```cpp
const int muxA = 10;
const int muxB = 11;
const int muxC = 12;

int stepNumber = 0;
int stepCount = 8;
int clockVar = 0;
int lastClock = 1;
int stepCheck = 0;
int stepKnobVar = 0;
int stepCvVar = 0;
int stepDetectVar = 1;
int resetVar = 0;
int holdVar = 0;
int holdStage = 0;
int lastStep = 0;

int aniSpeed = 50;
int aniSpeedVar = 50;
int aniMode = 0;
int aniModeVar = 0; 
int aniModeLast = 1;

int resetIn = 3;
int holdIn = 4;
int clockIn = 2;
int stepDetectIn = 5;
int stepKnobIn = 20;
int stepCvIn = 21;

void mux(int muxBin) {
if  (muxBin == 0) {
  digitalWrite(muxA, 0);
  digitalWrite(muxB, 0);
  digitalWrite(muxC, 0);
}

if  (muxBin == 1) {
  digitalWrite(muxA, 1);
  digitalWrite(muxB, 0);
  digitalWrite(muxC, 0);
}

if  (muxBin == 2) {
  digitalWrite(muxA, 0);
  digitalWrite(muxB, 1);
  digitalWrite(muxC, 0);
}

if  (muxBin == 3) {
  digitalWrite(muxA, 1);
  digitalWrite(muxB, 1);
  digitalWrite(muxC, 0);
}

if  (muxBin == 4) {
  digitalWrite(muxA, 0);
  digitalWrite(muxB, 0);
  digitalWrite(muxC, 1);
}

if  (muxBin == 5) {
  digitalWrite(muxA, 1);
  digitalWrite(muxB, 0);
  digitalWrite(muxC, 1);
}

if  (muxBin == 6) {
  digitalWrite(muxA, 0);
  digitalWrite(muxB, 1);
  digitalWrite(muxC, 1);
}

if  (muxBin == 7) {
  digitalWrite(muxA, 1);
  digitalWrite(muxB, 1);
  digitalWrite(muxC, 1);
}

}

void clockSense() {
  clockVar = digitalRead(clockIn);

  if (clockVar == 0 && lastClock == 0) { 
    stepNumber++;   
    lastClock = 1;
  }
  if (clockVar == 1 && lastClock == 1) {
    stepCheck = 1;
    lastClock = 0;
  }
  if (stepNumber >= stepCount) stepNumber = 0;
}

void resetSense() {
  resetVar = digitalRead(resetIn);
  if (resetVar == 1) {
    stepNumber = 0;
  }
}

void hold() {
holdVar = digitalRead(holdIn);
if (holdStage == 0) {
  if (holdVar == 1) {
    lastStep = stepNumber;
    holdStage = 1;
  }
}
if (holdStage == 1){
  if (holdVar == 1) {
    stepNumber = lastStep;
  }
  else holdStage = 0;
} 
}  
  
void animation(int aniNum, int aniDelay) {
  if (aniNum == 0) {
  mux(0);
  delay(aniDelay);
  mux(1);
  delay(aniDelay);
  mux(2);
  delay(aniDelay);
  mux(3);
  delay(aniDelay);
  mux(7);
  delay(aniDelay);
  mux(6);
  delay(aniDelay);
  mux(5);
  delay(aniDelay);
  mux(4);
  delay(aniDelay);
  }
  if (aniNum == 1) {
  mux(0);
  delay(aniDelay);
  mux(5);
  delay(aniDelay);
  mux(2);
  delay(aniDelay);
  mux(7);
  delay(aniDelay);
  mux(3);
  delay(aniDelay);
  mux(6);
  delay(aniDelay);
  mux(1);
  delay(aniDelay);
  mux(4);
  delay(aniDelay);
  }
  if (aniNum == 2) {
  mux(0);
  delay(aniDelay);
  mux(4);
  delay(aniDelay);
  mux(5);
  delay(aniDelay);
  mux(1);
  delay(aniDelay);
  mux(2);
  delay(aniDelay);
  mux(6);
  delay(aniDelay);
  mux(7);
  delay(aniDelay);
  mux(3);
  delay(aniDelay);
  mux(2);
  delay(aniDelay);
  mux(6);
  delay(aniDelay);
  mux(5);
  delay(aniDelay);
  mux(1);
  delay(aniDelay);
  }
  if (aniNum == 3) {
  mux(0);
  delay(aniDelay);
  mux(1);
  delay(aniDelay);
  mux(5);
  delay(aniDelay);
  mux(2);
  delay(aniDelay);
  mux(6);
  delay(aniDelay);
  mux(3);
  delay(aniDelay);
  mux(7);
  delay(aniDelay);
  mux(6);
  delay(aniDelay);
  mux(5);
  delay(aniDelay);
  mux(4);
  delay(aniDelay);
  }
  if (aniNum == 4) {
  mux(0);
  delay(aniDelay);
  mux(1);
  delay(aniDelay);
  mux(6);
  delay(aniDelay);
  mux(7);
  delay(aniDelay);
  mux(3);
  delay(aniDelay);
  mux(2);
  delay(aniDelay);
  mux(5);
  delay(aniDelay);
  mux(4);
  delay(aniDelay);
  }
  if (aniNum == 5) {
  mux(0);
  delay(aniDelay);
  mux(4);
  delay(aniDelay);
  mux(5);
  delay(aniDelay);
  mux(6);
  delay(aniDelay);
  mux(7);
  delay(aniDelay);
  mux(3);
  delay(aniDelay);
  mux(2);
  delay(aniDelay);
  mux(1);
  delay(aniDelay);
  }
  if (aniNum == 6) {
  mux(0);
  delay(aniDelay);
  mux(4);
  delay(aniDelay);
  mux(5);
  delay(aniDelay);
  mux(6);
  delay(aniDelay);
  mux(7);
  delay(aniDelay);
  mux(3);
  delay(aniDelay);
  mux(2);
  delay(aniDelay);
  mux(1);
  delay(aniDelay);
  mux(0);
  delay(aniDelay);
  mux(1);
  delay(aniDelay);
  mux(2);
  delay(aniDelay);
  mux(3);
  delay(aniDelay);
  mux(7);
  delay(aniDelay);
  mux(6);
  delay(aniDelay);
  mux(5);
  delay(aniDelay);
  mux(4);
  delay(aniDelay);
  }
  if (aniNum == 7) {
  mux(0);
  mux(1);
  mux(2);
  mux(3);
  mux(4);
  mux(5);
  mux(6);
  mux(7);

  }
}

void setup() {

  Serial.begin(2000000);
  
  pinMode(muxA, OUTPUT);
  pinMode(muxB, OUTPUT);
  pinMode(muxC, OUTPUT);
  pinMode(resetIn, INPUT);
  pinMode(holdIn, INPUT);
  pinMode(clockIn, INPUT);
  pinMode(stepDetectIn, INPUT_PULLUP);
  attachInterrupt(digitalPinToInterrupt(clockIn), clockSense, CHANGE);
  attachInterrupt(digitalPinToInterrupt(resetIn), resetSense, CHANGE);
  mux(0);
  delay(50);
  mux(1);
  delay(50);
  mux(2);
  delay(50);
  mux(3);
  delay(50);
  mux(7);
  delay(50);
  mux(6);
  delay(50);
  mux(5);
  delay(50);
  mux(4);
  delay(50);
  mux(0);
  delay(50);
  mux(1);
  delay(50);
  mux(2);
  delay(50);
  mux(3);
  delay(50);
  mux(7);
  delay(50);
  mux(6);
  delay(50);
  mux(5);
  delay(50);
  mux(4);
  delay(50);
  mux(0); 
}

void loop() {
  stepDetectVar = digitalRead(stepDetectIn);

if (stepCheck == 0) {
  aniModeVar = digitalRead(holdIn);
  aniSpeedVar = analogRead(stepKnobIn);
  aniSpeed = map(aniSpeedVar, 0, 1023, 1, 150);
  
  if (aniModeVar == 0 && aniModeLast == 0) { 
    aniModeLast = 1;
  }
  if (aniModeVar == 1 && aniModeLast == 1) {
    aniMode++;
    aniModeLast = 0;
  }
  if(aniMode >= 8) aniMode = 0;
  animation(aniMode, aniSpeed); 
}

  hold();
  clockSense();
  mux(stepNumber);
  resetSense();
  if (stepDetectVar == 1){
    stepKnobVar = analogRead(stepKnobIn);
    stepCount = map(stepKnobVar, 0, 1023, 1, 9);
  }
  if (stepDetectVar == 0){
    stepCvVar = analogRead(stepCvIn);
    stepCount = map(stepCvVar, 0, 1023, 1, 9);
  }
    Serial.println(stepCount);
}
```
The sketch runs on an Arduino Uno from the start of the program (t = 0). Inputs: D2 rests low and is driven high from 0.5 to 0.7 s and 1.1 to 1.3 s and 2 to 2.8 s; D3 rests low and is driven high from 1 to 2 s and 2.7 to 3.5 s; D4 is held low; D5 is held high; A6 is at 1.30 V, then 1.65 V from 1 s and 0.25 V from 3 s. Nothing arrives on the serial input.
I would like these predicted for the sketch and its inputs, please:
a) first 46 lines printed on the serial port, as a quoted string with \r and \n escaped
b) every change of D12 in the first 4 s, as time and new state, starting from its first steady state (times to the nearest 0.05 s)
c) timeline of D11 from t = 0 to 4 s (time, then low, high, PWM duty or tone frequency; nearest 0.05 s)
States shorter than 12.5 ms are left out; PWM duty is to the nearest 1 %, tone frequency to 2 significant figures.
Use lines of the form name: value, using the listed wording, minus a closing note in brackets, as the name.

first 46 lines printed on the serial port, as a quoted string with \r and \n escaped: "3\r\n3\r\n3\r\n3\r\n3\r\n3\r\n3\r\n3\r\n3\r\n3\r\n3\r\n3\r\n3\r\n3\r\n3\r\n3\r\n3\r\n3\r\n3\r\n3\r\n3\r\n3\r\n3\r\n3\r\n3\r\n3\r\n3\r\n3\r\n3\r\n3\r\n3\r\n3\r\n3\r\n3\r\n3\r\n3\r\n3\r\n3\r\n3\r\n3\r\n3\r\n3\r\n3\r\n3\r\n3\r\n3\r\n"
every change of D12 in the first 4 s, as time and new state, starting from its first steady state: 0 s low; 0.2 s high; 0.4 s low; 0.6 s high; 0.8 s low
timeline of D11 from t = 0 to 4 s: 0 s low; 0.1 s high; 0.3 s low; 0.5 s high; 0.7 s low
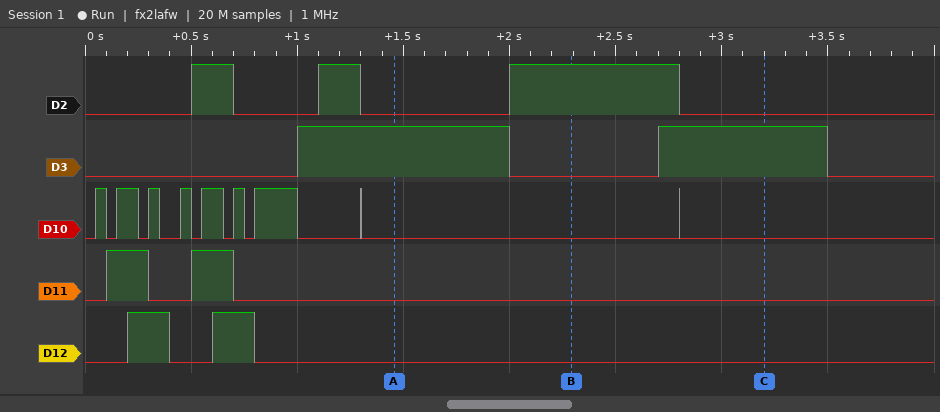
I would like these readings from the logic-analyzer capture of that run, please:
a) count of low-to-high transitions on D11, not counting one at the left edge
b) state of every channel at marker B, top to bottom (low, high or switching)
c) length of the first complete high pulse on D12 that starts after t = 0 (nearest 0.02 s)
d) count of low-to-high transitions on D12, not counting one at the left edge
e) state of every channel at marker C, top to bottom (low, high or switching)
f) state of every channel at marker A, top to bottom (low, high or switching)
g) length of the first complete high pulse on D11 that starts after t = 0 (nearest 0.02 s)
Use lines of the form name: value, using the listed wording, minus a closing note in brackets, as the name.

count of low-to-high transitions on D11, not counting one at the left edge: 2
state of every channel at marker B, top to bottom: D2 high, D3 low, D10 low, D11 low, D12 low
length of the first complete high pulse on D12 that starts after t = 0: 0.20 s
count of low-to-high transitions on D12, not counting one at the left edge: 2
state of every channel at marker C, top to bottom: D2 low, D3 high, D10 low, D11 low, D12 low
state of every channel at marker A, top to bottom: D2 low, D3 high, D10 low, D11 low, D12 low
length of the first complete high pulse on D11 that starts after t = 0: 0.20 s
